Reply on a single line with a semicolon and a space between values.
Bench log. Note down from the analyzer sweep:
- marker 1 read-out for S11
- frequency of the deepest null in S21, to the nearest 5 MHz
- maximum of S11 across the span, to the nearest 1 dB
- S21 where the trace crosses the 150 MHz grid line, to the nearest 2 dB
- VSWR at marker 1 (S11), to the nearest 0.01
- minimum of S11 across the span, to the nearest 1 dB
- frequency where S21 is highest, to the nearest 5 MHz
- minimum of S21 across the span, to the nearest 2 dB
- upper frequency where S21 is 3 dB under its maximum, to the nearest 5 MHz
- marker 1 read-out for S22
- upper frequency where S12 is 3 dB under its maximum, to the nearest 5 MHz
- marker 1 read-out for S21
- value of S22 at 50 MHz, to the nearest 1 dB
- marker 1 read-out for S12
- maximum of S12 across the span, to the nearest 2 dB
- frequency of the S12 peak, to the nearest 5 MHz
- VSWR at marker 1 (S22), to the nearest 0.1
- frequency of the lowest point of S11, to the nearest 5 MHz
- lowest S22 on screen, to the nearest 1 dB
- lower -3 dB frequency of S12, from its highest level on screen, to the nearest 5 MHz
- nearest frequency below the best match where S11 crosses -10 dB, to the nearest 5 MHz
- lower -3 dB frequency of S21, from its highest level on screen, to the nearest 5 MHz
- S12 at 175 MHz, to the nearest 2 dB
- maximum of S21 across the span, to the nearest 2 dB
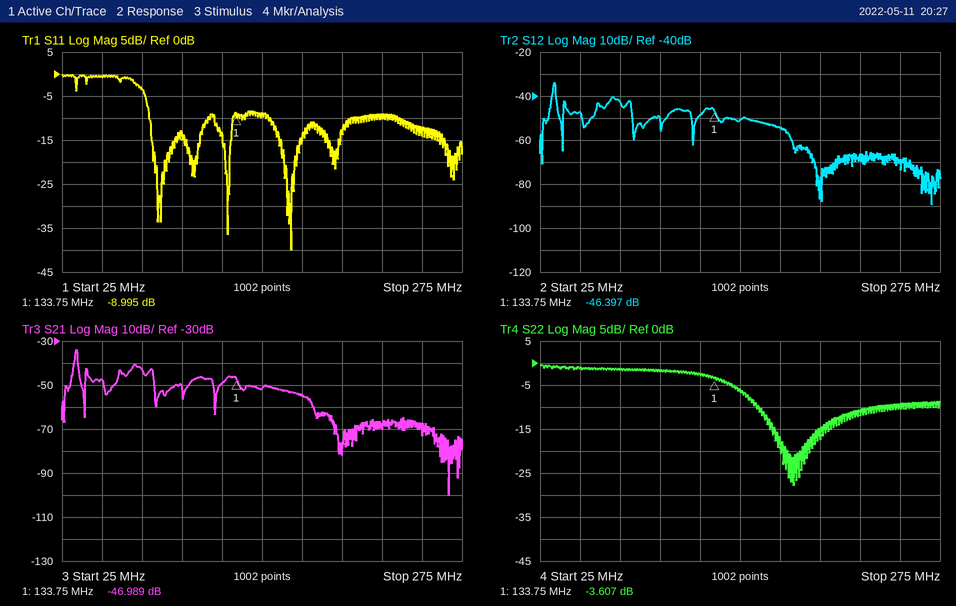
-8.995 dB; 265 MHz; 0 dB; -52 dB; 2.10; -40 dB; 35 MHz; -100 dB; 35 MHz; -3.607 dB; 35 MHz; -46.989 dB; -1 dB; -46.397 dB; -34 dB; 35 MHz; 4.9; 170 MHz; -28 dB; 35 MHz; 155 MHz; 35 MHz; -54 dB; -34 dB
